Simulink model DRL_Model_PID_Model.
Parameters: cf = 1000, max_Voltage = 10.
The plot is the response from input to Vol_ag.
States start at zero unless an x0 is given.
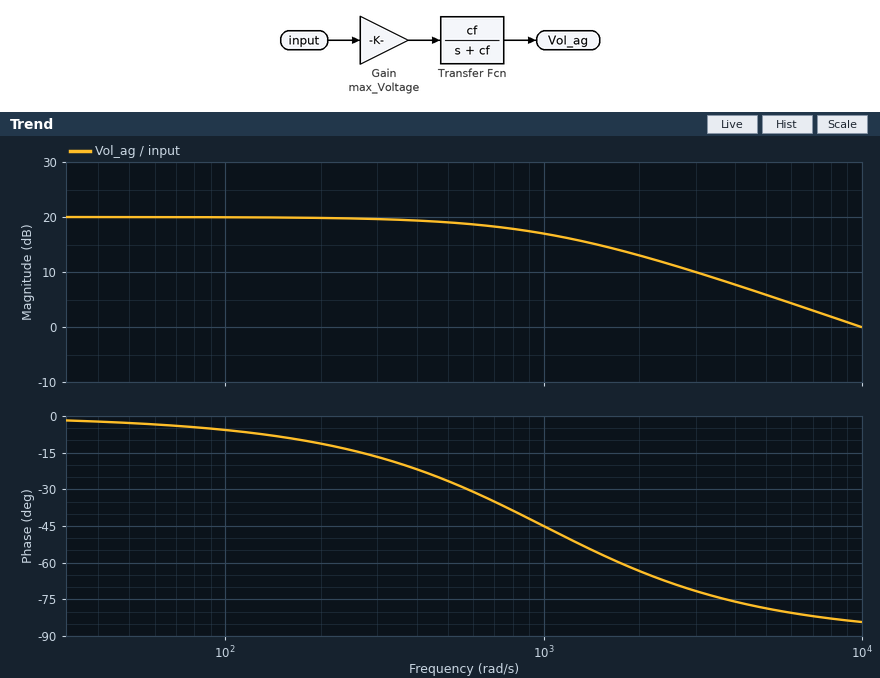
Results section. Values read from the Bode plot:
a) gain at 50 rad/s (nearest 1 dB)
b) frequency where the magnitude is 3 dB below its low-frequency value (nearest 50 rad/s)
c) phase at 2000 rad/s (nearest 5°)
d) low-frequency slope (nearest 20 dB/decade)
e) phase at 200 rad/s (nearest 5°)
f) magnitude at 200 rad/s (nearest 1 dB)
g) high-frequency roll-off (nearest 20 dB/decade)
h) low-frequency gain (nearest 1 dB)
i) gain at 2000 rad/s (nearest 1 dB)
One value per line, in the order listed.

20 dB
1000 rad/s
-65°
0 dB/decade
-10°
20 dB
-20 dB/decade
20 dB
13 dB
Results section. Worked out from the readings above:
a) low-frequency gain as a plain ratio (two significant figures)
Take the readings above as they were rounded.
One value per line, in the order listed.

10
